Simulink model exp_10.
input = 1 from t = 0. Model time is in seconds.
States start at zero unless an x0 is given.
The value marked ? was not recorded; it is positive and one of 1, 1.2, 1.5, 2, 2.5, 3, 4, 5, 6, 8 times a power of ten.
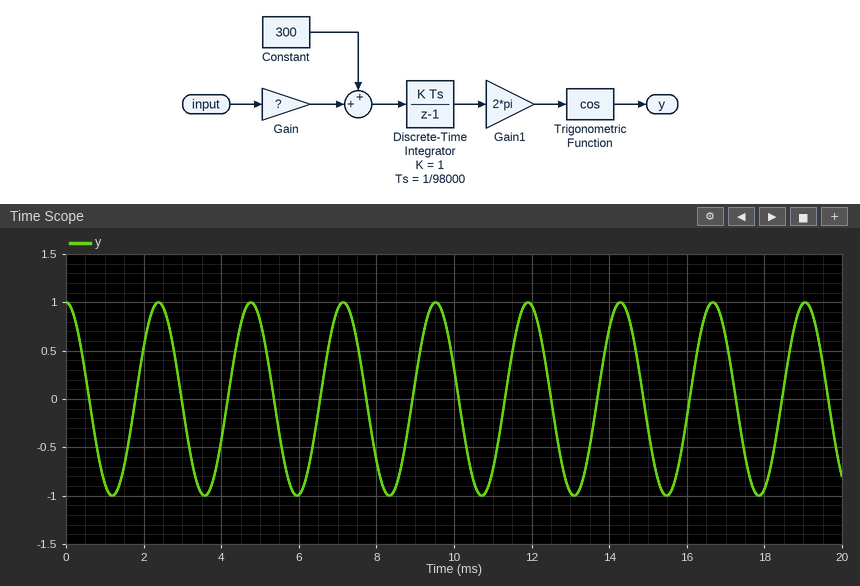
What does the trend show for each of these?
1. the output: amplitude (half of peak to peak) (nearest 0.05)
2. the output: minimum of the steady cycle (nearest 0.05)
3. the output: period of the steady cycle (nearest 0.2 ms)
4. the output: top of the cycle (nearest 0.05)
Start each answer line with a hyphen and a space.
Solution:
- 1.00
- -1.00
- 2.4 ms
- 1.00
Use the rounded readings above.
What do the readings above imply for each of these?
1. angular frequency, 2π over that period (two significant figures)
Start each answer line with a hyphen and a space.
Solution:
- 2.6 rad/ms
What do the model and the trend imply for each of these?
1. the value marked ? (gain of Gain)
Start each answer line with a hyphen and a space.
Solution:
- 120
